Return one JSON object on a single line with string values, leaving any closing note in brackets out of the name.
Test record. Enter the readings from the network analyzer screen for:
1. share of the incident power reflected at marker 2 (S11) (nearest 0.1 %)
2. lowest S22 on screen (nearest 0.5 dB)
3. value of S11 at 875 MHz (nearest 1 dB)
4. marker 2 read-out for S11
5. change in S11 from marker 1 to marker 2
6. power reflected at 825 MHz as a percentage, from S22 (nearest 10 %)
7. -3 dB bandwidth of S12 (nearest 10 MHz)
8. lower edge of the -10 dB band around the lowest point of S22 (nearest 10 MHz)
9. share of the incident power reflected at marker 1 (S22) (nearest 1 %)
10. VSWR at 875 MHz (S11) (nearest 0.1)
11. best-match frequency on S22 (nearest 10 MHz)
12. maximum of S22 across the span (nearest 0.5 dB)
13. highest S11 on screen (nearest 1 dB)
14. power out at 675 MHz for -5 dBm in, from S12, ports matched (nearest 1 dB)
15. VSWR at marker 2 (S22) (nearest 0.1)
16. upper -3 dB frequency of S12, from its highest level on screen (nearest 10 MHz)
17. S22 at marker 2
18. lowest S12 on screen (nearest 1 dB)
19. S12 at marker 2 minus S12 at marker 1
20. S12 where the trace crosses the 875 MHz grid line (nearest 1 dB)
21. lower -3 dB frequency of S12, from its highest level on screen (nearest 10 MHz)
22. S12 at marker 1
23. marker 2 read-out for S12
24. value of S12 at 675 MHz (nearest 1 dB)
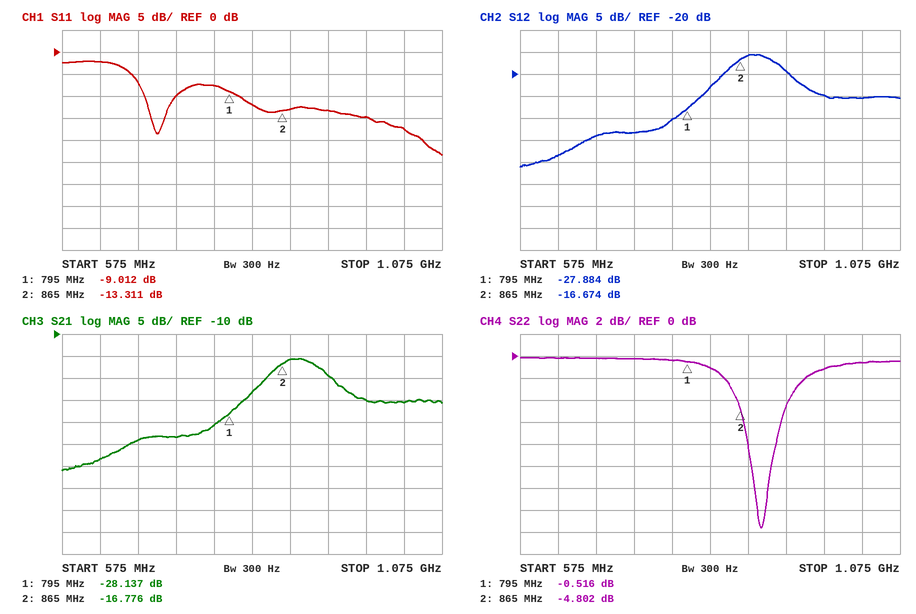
{"share of the incident power reflected at marker 2 (S11)": "4.7 %", "lowest S22 on screen": "-15.5 dB", "value of S11 at 875 MHz": "-13 dB", "marker 2 read-out for S11": "-13.311 dB", "change in S11 from marker 1 to marker 2": "-4.299 dB", "power reflected at 825 MHz as a percentage, from S22": "80 %", "-3 dB bandwidth of S12": "70 MHz", "lower edge of the -10 dB band around the lowest point of S22": "880 MHz", "share of the incident power reflected at marker 1 (S22)": "89 %", "VSWR at 875 MHz (S11)": "1.6", "best-match frequency on S22": "890 MHz", "maximum of S22 across the span": "0.0 dB", "highest S11 on screen": "-2 dB", "power out at 675 MHz for -5 dBm in, from S12, ports matched": "-39 dBm", "VSWR at marker 2 (S22)": "3.7", "upper -3 dB frequency of S12, from its highest level on screen": "920 MHz", "S22 at marker 2": "-4.802 dB", "lowest S12 on screen": "-41 dB", "S12 at marker 2 minus S12 at marker 1": "11.210 dB", "S12 where the trace crosses the 875 MHz grid line": "-16 dB", "lower -3 dB frequency of S12, from its highest level on screen": "850 MHz", "S12 at marker 1": "-27.884 dB", "marker 2 read-out for S12": "-16.674 dB", "value of S12 at 675 MHz": "-34 dB"}
